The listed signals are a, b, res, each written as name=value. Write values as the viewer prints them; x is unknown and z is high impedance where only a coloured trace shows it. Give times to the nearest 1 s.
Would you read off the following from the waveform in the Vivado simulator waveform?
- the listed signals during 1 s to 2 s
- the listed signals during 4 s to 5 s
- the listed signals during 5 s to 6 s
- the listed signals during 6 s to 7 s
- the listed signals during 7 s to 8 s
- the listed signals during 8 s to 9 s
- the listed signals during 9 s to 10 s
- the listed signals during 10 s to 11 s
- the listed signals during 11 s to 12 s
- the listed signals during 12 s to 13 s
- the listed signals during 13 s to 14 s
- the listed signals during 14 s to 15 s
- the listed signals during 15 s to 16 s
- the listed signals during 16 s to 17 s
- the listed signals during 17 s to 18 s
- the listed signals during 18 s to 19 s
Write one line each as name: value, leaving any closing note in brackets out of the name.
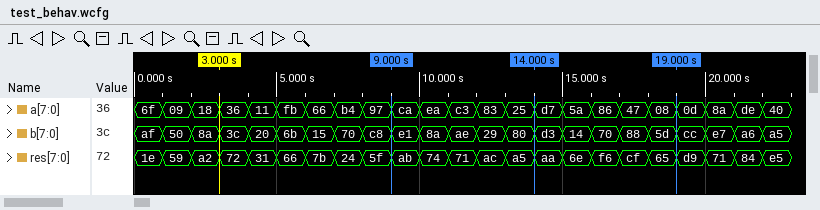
the listed signals during 1 s to 2 s: a=09, b=50, res=59
the listed signals during 4 s to 5 s: a=11, b=20, res=31
the listed signals during 5 s to 6 s: a=fb, b=6b, res=66
the listed signals during 6 s to 7 s: a=66, b=15, res=7b
the listed signals during 7 s to 8 s: a=b4, b=70, res=24
the listed signals during 8 s to 9 s: a=97, b=c8, res=5f
the listed signals during 9 s to 10 s: a=ca, b=e1, res=ab
the listed signals during 10 s to 11 s: a=ea, b=8a, res=74
the listed signals during 11 s to 12 s: a=c3, b=ae, res=71
the listed signals during 12 s to 13 s: a=83, b=29, res=ac
the listed signals during 13 s to 14 s: a=25, b=80, res=a5
the listed signals during 14 s to 15 s: a=d7, b=d3, res=aa
the listed signals during 15 s to 16 s: a=5a, b=14, res=6e
the listed signals during 16 s to 17 s: a=86, b=70, res=f6
the listed signals during 17 s to 18 s: a=47, b=88, res=cf
the listed signals during 18 s to 19 s: a=08, b=5d, res=65
